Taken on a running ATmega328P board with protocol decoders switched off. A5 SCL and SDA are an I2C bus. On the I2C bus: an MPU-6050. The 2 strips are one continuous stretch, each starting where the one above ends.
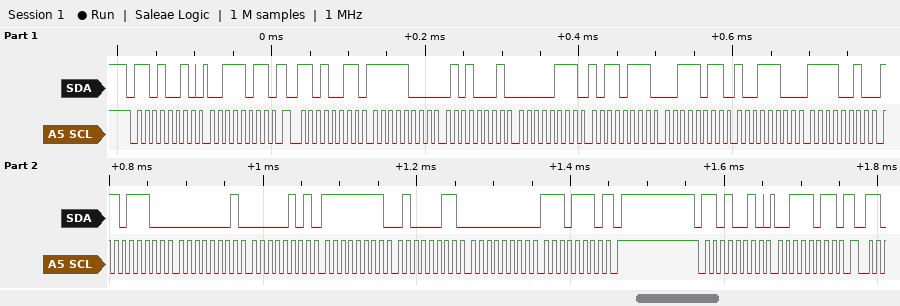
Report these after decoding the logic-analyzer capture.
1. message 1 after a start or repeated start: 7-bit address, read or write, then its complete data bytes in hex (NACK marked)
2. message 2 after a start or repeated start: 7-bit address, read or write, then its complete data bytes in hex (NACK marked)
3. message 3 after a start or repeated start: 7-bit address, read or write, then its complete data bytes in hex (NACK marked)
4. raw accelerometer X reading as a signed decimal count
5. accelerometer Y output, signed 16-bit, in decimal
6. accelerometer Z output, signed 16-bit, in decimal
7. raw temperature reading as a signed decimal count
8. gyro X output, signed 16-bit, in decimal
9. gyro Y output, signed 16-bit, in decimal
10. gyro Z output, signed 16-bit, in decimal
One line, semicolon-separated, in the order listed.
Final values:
0x69 write: 3B; 0x69 read: F8 51 07 B7 3B 9C F2 DC 01 05 FF 43 00 EE NACK; 0x69 write: 3B; -1967; 1975; 15260; -3364; 261; -189; 238
